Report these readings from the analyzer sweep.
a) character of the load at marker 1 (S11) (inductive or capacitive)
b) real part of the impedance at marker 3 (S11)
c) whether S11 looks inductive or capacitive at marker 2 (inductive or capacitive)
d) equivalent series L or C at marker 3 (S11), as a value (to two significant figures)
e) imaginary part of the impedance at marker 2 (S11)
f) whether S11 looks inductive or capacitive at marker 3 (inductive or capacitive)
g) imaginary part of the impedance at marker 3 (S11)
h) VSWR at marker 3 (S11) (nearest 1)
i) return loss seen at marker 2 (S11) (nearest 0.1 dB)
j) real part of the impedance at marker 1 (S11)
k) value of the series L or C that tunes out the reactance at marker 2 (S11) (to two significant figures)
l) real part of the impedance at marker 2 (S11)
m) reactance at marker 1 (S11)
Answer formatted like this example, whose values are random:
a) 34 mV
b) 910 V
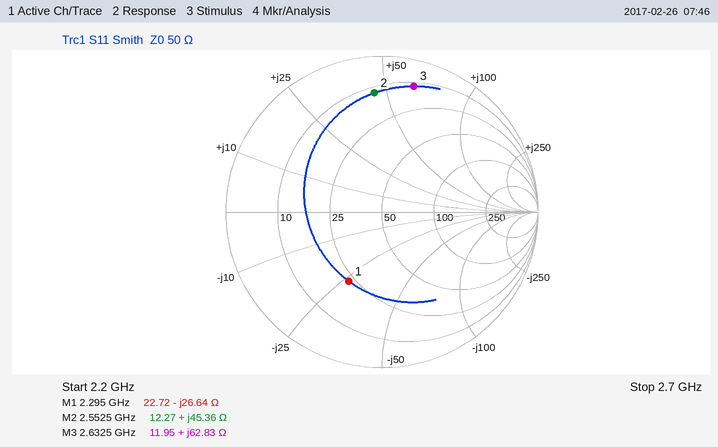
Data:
a) capacitive
b) 11.95 Ω
c) inductive
d) 3.8 nH
e) +45.36 Ω
f) inductive
g) +62.83 Ω
h) 11
i) 2.3 dB
j) 22.72 Ω
k) 1.4 pF
l) 12.27 Ω
m) -26.64 Ω
